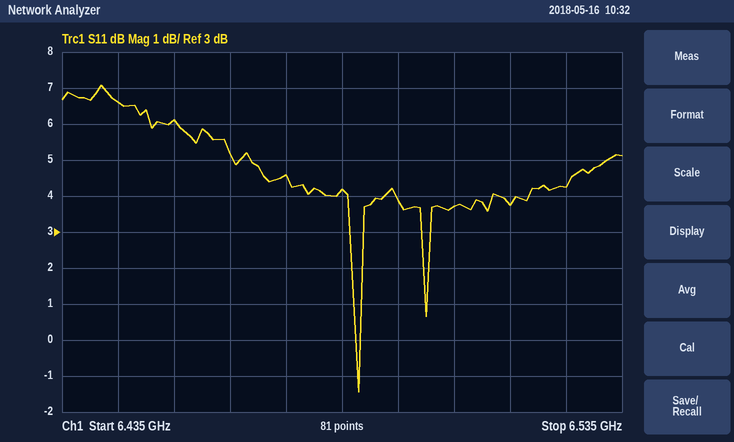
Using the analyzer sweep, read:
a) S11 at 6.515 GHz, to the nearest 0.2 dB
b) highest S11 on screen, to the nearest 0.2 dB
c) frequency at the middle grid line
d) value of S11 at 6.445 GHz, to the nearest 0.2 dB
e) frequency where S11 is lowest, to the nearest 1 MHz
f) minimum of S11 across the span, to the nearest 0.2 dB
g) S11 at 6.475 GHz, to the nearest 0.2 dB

3.8 dB
7.0 dB
6.485 GHz
6.6 dB
6.488 GHz
-1.4 dB
4.6 dB
